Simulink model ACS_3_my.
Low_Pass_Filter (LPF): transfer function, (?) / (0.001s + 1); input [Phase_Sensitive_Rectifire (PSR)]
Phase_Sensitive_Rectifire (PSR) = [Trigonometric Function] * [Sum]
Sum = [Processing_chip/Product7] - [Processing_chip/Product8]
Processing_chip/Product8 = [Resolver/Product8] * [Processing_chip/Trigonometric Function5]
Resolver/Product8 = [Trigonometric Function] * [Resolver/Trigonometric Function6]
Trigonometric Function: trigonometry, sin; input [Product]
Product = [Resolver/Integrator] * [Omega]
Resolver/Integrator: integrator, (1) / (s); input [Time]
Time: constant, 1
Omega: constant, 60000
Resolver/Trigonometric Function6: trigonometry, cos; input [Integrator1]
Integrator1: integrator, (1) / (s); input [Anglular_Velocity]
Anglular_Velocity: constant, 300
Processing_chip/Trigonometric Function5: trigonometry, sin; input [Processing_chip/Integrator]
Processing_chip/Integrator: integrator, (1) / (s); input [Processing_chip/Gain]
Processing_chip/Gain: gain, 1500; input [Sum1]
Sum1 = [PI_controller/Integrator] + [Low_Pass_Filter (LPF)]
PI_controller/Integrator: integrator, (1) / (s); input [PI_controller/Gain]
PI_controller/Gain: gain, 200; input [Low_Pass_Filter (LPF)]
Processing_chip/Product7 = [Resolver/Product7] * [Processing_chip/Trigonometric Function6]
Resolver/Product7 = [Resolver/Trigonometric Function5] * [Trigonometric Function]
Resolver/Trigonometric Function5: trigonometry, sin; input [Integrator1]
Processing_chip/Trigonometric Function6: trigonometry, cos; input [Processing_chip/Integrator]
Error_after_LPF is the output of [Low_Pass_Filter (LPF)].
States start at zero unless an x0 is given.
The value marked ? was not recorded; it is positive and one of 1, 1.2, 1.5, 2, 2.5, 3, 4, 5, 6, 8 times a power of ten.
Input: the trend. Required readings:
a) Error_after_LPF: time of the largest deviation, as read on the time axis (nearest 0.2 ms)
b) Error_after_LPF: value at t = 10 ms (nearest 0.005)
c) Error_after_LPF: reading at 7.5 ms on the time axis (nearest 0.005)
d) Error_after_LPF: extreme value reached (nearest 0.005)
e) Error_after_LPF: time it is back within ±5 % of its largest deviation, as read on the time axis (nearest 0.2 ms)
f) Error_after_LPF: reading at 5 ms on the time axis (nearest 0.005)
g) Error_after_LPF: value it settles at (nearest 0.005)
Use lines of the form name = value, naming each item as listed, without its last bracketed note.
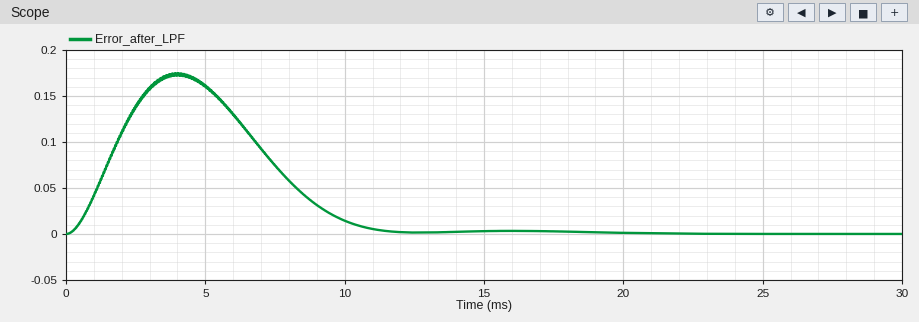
Error_after_LPF: time of the largest deviation, as read on the time axis = 4.0 ms
Error_after_LPF: value at t = 10 ms = 0.015
Error_after_LPF: reading at 7.5 ms on the time axis = 0.075
Error_after_LPF: extreme value reached = 0.175
Error_after_LPF: time it is back within ±5 % of its largest deviation, as read on the time axis = 10.6 ms
Error_after_LPF: reading at 5 ms on the time axis = 0.160
Error_after_LPF: value it settles at = 0.000
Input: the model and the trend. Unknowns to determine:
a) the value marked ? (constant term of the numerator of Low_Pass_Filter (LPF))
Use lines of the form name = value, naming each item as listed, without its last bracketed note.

the value marked ? (constant term of the numerator of Low_Pass_Filter (LPF)) = 0.8
